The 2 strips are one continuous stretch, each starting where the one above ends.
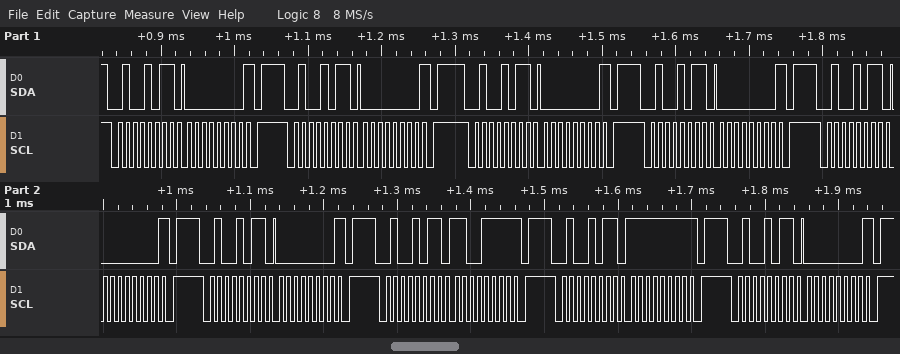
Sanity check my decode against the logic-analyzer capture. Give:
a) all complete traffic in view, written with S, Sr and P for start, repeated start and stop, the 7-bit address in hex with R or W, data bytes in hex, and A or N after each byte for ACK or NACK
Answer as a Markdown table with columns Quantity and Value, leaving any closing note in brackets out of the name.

| Quantity | Value |
|---|---|
| all complete traffic in view, written with S, Sr and P for start, repeated start and stop, the 7-bit address in hex with R or W, data bytes in hex, and A or N after each byte for ACK or NACK | S 25R A 00 N P S 25R A 00 N P S 25R A 00 N P S 25R A 00 N P S 25R A 00 N P S 25R A 00 N P S 25R A CF N P S 25R A FF N P S 25R A 00 N P |
